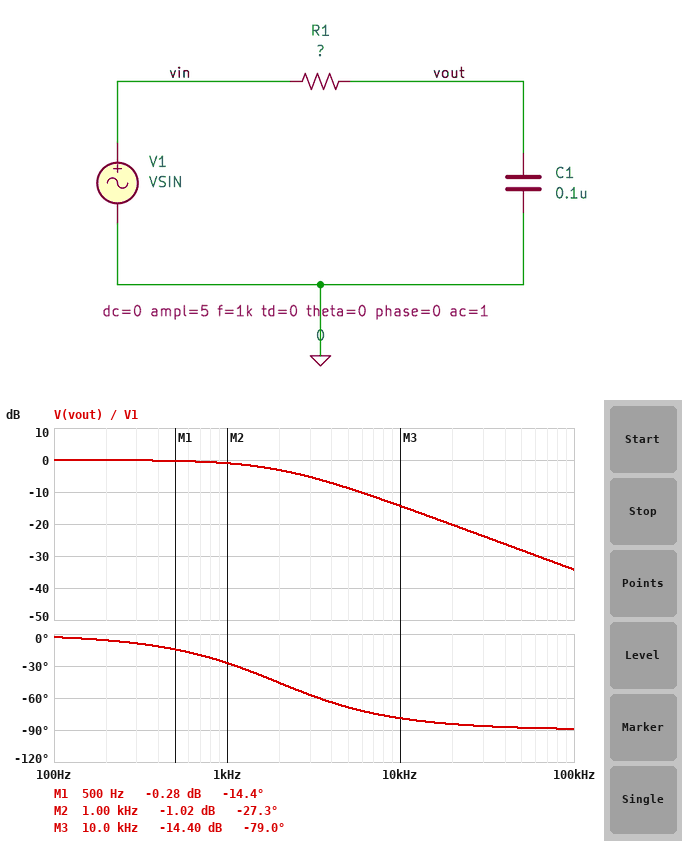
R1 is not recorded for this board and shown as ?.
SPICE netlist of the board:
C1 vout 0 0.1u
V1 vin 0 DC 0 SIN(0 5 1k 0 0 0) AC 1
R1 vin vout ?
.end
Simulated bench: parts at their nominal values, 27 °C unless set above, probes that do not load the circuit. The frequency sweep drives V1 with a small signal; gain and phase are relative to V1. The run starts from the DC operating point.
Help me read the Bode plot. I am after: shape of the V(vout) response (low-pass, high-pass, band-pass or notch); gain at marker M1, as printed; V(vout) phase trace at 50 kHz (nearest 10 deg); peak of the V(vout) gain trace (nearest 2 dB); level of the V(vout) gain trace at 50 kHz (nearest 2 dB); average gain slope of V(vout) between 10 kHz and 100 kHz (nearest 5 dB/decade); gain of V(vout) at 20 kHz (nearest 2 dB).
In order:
low-pass
-0.28 dB
-90 deg
0 dB
-28 dB
-20 dB/decade
-20 dB
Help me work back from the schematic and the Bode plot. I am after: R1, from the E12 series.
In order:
820 Ω
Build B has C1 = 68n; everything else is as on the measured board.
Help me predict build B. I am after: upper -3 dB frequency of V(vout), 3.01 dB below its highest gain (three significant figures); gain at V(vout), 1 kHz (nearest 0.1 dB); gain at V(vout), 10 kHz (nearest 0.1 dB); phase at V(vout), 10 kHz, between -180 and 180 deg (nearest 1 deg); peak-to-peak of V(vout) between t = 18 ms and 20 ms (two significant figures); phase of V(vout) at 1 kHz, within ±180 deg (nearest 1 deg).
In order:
2.85 kHz
-0.5 dB
-11.2 dB
-74 deg
9.4 V
-19 deg
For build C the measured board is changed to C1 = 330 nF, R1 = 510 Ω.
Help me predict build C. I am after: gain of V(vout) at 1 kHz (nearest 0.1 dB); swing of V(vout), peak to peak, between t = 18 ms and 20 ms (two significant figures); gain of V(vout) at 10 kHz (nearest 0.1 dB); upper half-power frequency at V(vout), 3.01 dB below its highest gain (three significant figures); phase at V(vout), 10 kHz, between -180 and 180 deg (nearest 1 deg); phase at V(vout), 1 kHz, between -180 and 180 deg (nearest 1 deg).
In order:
-3.3 dB
6.9 V
-20.5 dB
946 Hz
-85 deg
-47 deg
